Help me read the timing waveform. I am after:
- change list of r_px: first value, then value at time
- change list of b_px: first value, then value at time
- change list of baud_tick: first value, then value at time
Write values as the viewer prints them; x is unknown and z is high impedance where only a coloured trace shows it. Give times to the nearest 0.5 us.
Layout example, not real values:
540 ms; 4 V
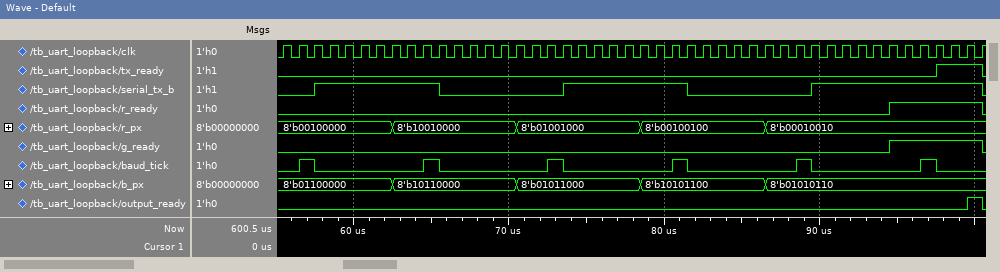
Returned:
8'b00100000, 8'b10010000 at 62.5 us, 8'b01001000 at 70.5 us, 8'b00100100 at 78.5 us, 8'b00010010 at 86.5 us; 8'b01100000, 8'b10110000 at 62.5 us, 8'b01011000 at 70.5 us, 8'b10101100 at 78.5 us, 8'b01010110 at 86.5 us; 0, 1 at 56.5 us, 0 at 57.5 us, 1 at 64.5 us, 0 at 65.5 us, 1 at 72.5 us, 0 at 73.5 us, 1 at 80.5 us, 0 at 81.5 us, 1 at 88.5 us, 0 at 89.5 us, 1 at 96.5 us, 0 at 97.5 us
